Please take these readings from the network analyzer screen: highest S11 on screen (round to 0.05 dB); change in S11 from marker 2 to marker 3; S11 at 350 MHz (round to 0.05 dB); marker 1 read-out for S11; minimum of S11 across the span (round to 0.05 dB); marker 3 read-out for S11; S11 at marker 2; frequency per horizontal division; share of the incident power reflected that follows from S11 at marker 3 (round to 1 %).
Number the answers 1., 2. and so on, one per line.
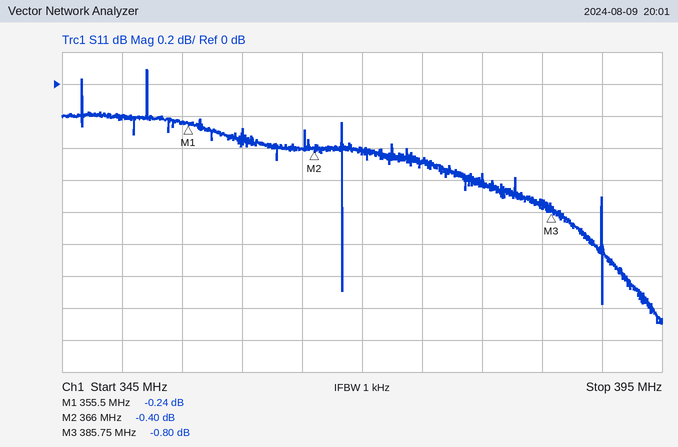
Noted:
1. 0.10 dB
2. -0.40 dB
3. -0.20 dB
4. -0.24 dB
5. -1.50 dB
6. -0.80 dB
7. -0.40 dB
8. 5 MHz
9. 83 %
